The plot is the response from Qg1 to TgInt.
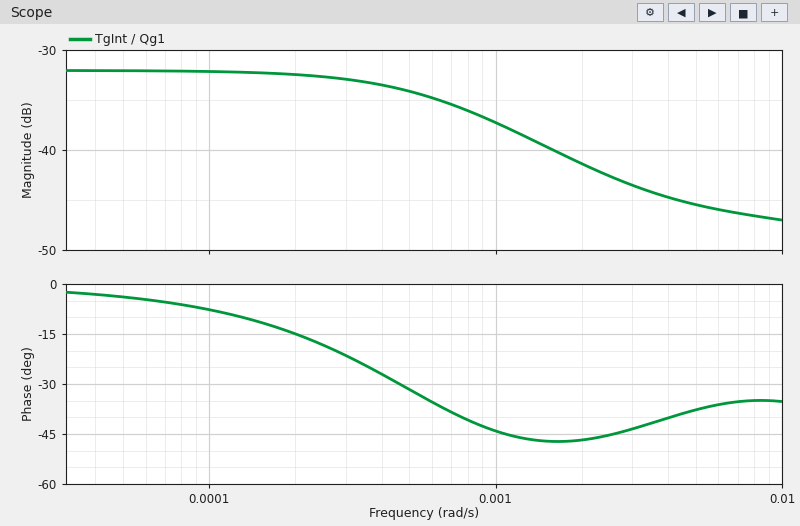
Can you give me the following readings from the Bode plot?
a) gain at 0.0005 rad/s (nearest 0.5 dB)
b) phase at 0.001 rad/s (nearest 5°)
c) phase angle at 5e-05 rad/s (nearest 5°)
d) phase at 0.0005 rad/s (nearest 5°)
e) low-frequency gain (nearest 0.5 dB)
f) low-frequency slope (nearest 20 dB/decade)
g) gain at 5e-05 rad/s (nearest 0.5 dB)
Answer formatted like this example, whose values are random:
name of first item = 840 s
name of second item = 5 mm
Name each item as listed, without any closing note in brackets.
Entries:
gain at 0.0005 rad/s = -34.0 dB
phase at 0.001 rad/s = -45°
phase angle at 5e-05 rad/s = -5°
phase at 0.0005 rad/s = -30°
low-frequency gain = -32.0 dB
low-frequency slope = 0 dB/decade
gain at 5e-05 rad/s = -32.0 dB
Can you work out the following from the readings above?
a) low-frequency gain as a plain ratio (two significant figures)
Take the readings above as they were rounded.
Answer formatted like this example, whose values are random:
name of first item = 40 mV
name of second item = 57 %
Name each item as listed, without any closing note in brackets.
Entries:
low-frequency gain as a plain ratio = 0.025
